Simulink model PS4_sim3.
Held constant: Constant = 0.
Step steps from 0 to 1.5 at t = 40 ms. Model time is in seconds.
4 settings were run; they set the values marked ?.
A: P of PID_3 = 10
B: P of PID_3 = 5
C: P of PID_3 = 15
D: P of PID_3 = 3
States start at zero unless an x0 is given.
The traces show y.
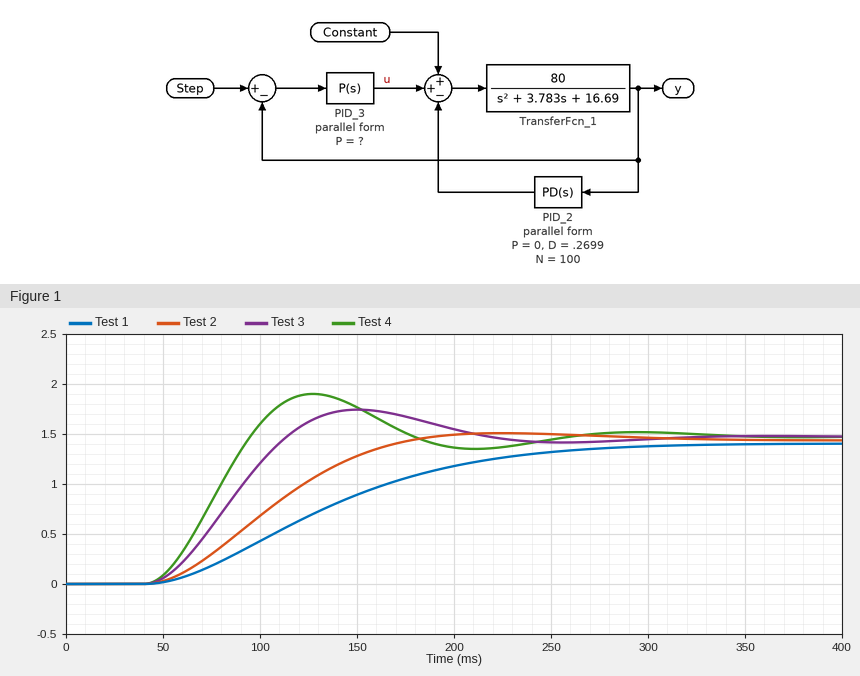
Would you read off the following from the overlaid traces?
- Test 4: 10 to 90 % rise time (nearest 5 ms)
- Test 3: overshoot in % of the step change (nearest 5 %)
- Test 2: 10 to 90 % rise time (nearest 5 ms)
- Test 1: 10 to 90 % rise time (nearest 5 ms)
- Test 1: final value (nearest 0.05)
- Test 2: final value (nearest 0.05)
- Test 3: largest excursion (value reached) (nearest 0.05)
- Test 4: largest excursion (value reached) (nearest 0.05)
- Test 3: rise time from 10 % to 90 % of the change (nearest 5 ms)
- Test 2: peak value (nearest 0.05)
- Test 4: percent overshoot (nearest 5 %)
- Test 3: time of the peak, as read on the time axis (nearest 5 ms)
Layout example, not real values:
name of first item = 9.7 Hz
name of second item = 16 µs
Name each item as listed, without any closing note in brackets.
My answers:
Test 4: 10 to 90 % rise time = 35 ms
Test 3: overshoot in % of the step change = 20 %
Test 2: 10 to 90 % rise time = 90 ms
Test 1: 10 to 90 % rise time = 155 ms
Test 1: final value = 1.40
Test 2: final value = 1.45
Test 3: largest excursion (value reached) = 1.75
Test 4: largest excursion (value reached) = 1.90
Test 3: rise time from 10 % to 90 % of the change = 50 ms
Test 2: peak value = 1.50
Test 4: percent overshoot = 30 %
Test 3: time of the peak, as read on the time axis = 150 ms
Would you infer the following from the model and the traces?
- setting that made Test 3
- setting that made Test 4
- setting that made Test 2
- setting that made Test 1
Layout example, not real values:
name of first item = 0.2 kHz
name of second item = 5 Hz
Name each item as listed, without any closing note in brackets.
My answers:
setting that made Test 3 = A
setting that made Test 4 = C
setting that made Test 2 = B
setting that made Test 1 = D
